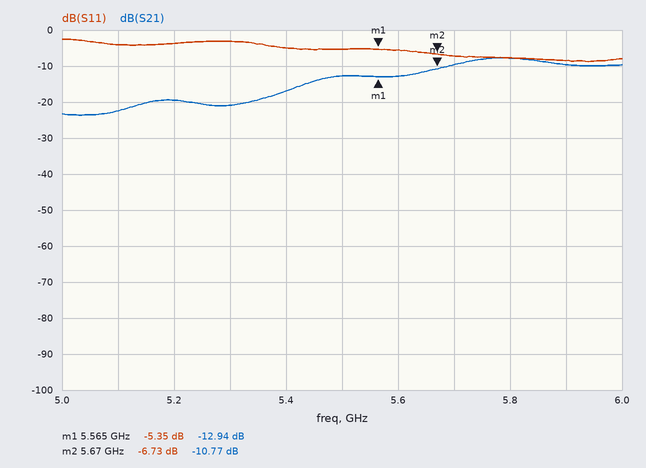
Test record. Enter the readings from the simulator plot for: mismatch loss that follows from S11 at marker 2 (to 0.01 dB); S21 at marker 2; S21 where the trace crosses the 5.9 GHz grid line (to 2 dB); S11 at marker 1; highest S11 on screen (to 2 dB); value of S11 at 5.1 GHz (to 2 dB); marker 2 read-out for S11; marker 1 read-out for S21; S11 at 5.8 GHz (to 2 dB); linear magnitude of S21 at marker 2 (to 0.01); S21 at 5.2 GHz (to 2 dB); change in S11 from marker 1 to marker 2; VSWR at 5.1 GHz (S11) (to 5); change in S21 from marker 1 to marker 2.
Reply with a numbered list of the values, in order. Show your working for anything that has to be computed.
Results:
1. −10 log10(1 − 10^(-6.73/10)) ≈ 1.04 dB
2. -10.77 dB
3. -10 dB
4. -5.35 dB
5. -2 dB
6. -4 dB
7. -6.73 dB
8. -12.94 dB
9. -8 dB
10. 10^(-10.77/20) ≈ 0.29
11. -20 dB
12. -6.73 − (-5.35) = -1.38 dB
13. |Γ| = 10^(-4/20) = 0.6310; VSWR = (1 + 0.6310)/(1 − 0.6310) ≈ 4.42, so 5 to the nearest 5
14. -10.77 − (-12.94) = 2.17 dB
